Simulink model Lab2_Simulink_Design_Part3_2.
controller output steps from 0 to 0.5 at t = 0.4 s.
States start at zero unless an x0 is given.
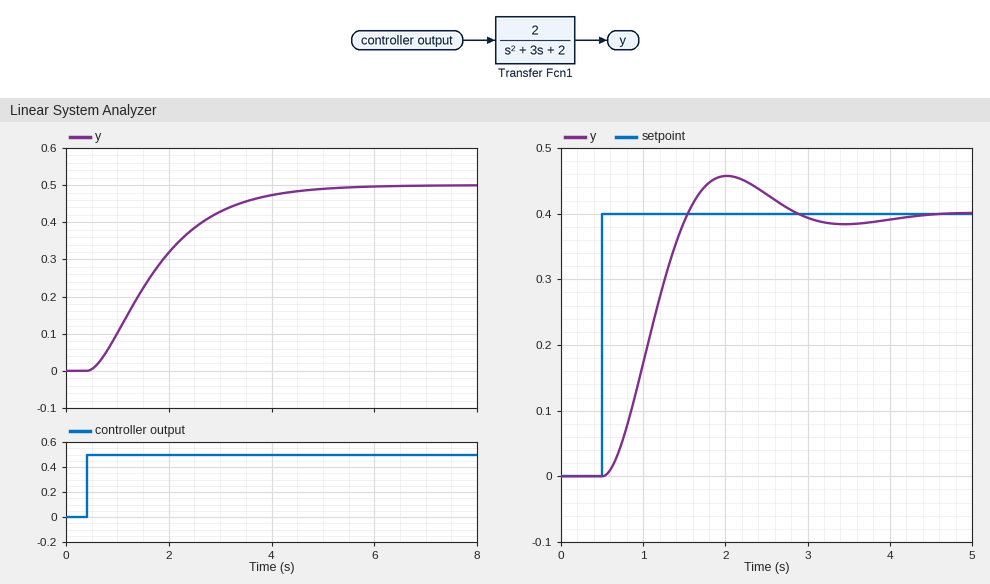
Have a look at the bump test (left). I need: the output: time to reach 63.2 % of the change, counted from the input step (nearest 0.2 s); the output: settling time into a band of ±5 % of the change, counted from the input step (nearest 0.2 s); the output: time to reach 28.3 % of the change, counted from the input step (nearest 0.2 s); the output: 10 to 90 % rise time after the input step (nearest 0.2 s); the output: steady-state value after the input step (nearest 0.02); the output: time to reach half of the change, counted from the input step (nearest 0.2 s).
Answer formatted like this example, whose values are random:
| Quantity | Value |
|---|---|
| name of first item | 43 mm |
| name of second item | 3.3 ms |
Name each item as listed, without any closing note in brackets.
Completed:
| Quantity | Value |
|---|---|
| the output: time to reach 63.2 % of the change, counted from the input step | 1.6 s |
| the output: settling time into a band of ±5 % of the change, counted from the input step | 3.6 s |
| the output: time to reach 28.3 % of the change, counted from the input step | 0.8 s |
| the output: 10 to 90 % rise time after the input step | 2.6 s |
| the output: steady-state value after the input step | 0.50 |
| the output: time to reach half of the change, counted from the input step | 1.2 s |
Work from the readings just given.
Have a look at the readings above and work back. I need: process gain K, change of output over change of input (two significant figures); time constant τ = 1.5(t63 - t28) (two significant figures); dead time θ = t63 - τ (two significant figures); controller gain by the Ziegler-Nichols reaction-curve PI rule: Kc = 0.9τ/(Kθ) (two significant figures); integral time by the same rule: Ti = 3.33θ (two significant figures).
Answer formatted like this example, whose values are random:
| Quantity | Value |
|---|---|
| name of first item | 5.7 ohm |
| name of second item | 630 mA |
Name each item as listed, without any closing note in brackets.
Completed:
| Quantity | Value |
|---|---|
| process gain K, change of output over change of input | 1.0 |
| time constant τ = 1.5(t63 - t28) | 1.2 s |
| dead time θ = t63 - τ | 0.40 s |
| controller gain by the Ziegler-Nichols reaction-curve PI rule: Kc = 0.9τ/(Kθ) | 2.7 |
| integral time by the same rule: Ti = 3.33θ | 1.3 s |
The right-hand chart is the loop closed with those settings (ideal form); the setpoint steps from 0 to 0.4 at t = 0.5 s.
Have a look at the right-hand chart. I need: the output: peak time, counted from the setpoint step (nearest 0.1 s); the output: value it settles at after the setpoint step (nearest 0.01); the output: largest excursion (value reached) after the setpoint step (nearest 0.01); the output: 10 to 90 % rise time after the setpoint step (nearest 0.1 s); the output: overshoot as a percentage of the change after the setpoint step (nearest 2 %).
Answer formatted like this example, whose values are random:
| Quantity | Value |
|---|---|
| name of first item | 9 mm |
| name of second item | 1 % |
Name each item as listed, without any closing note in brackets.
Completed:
| Quantity | Value |
|---|---|
| the output: peak time, counted from the setpoint step | 1.5 s |
| the output: value it settles at after the setpoint step | 0.40 |
| the output: largest excursion (value reached) after the setpoint step | 0.46 |
| the output: 10 to 90 % rise time after the setpoint step | 0.7 s |
| the output: overshoot as a percentage of the change after the setpoint step | 14 % |
